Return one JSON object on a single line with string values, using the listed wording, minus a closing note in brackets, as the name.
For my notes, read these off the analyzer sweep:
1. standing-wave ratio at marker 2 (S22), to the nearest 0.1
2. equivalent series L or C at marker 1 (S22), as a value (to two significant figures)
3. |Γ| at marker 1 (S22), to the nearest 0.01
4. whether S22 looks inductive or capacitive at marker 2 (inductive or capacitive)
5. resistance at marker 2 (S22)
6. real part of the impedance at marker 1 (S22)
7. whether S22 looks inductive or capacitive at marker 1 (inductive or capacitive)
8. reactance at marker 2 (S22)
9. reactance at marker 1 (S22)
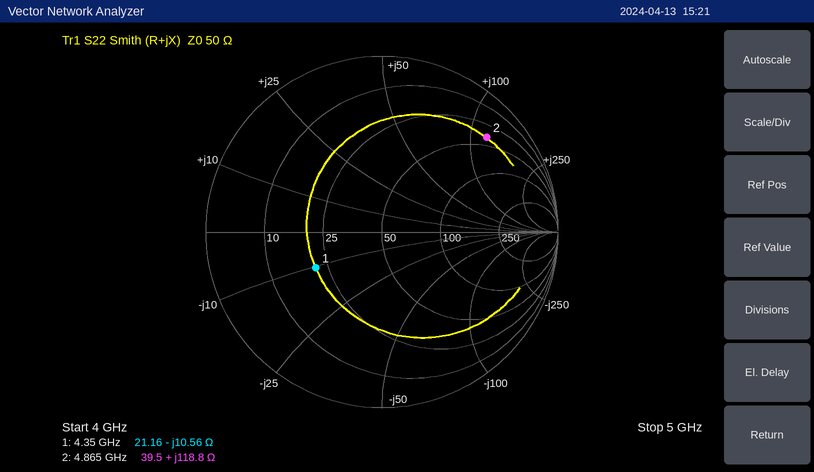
{"standing-wave ratio at marker 2 (S22), to the nearest 0.1": "9.1", "equivalent series L or C at marker 1 (S22), as a value": "3.5 pF", "|Γ| at marker 1 (S22), to the nearest 0.01": "0.43", "whether S22 looks inductive or capacitive at marker 2": "inductive", "resistance at marker 2": "39.5 Ω", "real part of the impedance at marker 1": "21.16 Ω", "whether S22 looks inductive or capacitive at marker 1": "capacitive", "reactance at marker 2": "+118.8 Ω", "reactance at marker 1": "-10.56 Ω"}
